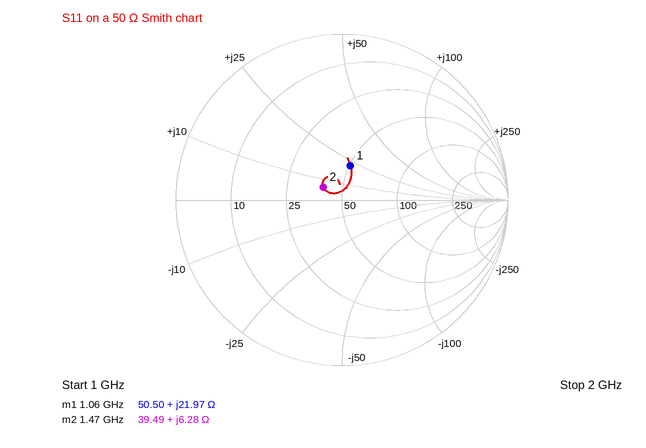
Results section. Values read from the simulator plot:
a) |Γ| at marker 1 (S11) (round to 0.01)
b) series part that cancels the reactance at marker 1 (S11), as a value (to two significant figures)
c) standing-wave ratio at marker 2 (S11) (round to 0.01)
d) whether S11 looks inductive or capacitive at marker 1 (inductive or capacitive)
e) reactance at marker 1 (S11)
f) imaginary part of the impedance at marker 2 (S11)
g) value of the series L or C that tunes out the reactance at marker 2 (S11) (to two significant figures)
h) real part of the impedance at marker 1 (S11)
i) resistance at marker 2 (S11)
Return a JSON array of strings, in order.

["0.21", "6.8 pF", "1.32", "inductive", "+21.97 Ω", "+6.28 Ω", "17 pF", "50.50 Ω", "39.49 Ω"]
